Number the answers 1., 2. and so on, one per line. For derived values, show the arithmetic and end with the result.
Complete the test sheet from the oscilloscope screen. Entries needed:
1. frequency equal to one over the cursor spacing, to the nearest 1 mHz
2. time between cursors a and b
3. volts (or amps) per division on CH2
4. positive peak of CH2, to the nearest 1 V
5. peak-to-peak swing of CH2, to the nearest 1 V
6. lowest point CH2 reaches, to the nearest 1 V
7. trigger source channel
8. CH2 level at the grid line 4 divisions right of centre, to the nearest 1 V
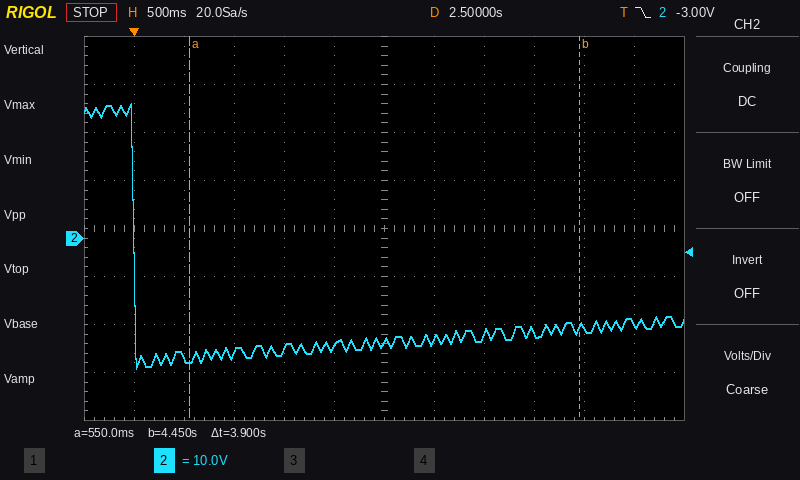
1. 1 / 3.9 s ≈ 256 mHz
2. 3.9 s
3. 10 V
4. 28 V
5. 28 V − (-27 V) = 55 V
6. -27 V
7. CH2
8. -19 V
